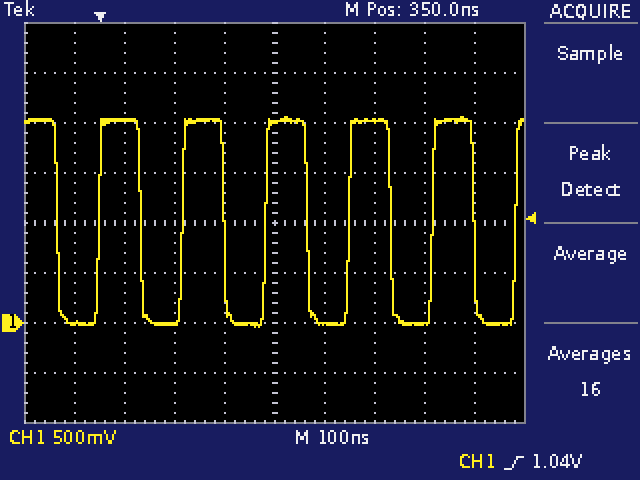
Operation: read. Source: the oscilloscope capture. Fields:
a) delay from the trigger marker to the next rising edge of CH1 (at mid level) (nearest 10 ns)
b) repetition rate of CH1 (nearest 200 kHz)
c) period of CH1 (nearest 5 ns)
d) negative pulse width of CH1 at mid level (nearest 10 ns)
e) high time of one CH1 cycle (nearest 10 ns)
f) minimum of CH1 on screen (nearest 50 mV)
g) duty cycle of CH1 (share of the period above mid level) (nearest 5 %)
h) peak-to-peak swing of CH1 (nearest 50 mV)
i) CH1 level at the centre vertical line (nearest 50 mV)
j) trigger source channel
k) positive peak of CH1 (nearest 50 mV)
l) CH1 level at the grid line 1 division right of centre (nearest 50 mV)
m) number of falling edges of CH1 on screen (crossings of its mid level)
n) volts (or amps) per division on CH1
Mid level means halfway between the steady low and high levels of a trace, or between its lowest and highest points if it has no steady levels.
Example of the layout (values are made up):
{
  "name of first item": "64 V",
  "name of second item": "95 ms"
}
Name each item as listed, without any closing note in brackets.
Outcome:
{
  "delay from the trigger marker to the next rising edge of CH1 (at mid level)": "170 ns",
  "repetition rate of CH1": "6.0 MHz",
  "period of CH1": "165 ns",
  "negative pulse width of CH1 at mid level": "80 ns",
  "high time of one CH1 cycle": "80 ns",
  "minimum of CH1 on screen": "-50 mV",
  "duty cycle of CH1 (share of the period above mid level)": "50 %",
  "peak-to-peak swing of CH1": "2.10 V",
  "CH1 level at the centre vertical line": "2.00 V",
  "trigger source channel": "CH1",
  "positive peak of CH1": "2.05 V",
  "CH1 level at the grid line 1 division right of centre": "0 mV",
  "number of falling edges of CH1 on screen": "6",
  "volts (or amps) per division on CH1": "500 mV"
}
